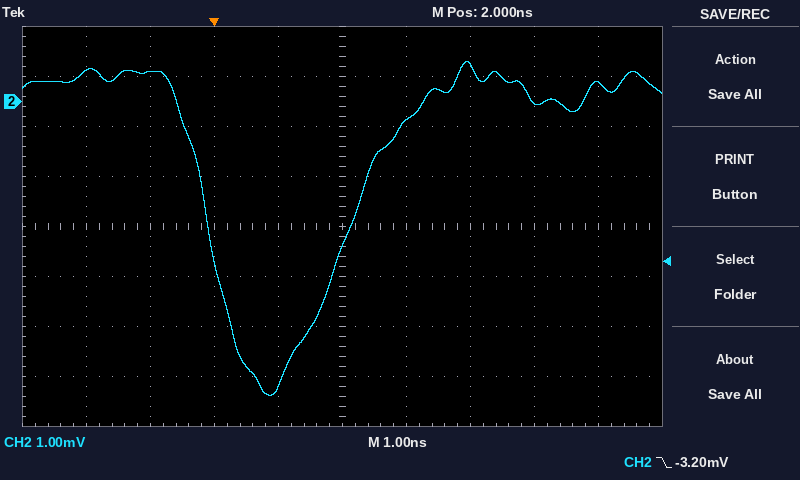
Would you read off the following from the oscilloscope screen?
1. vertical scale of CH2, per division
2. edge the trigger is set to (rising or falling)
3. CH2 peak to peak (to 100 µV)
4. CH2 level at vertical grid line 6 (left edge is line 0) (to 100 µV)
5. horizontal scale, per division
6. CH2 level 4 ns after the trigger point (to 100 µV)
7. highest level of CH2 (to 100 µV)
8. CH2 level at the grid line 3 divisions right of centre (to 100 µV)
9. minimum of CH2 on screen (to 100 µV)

1 mV
falling
6.7 mV
-400 µV
1 ns
700 µV
800 µV
0.0 mV
-5.9 mV
